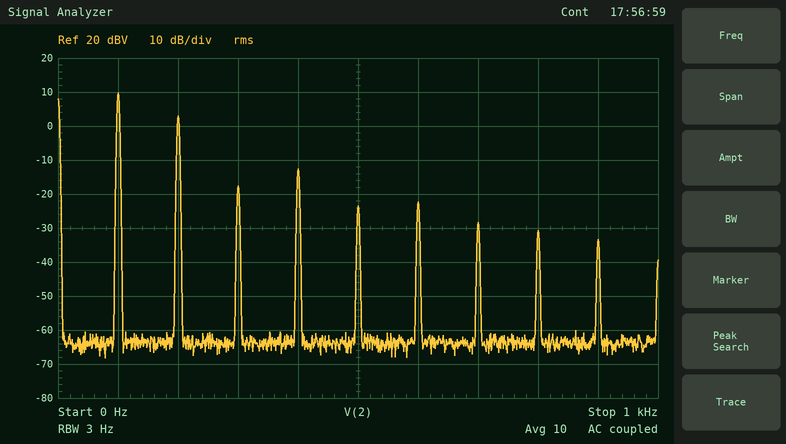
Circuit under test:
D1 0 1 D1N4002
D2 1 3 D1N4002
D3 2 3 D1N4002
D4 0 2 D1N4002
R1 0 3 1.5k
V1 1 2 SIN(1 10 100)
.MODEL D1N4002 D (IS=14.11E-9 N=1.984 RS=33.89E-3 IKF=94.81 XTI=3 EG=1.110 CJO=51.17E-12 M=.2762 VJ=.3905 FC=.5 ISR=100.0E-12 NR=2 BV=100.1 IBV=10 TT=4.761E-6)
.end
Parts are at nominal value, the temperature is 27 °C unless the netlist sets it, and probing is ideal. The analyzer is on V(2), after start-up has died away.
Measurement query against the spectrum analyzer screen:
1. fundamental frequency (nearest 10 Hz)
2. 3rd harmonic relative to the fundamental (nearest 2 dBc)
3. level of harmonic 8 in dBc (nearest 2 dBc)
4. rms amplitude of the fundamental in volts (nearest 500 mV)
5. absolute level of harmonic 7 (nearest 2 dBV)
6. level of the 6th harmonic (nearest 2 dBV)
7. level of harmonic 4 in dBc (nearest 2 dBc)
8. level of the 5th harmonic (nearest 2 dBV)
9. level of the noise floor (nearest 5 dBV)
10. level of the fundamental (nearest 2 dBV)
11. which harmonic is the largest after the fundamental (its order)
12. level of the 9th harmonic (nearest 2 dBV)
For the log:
100 Hz
-28 dBc
-40 dBc
3.0 V
-28 dBV
-22 dBV
-22 dBc
-24 dBV
-65 dBV
10 dBV
2
-34 dBV
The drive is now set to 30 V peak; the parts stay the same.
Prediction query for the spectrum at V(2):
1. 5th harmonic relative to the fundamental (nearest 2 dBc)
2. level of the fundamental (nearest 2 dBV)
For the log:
-42 dBc
20 dBV
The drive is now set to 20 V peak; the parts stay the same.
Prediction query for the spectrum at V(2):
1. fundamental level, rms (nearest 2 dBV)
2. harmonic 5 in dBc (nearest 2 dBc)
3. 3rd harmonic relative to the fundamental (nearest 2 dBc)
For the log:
16 dBV
-38 dBc
-34 dBc
